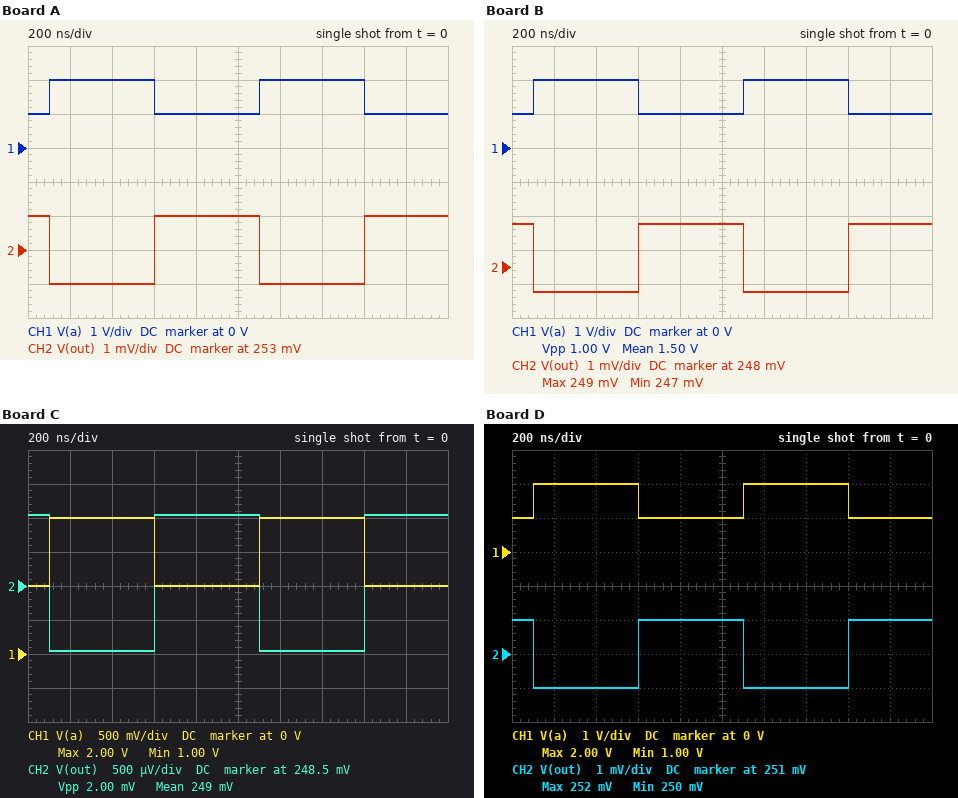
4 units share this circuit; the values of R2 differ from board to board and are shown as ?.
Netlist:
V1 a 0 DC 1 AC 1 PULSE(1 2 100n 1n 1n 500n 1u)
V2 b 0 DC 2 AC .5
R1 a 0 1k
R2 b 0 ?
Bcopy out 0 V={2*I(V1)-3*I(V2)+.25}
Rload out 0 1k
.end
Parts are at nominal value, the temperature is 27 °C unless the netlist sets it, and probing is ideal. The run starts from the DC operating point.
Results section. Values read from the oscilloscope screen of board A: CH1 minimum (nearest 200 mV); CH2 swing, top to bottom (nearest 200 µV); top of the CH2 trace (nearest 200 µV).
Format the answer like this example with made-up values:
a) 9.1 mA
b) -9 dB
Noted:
a) 1.0 V
b) 2.0 mV
c) 254.0 mV
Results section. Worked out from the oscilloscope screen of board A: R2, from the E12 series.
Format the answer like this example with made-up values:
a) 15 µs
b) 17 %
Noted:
a) 1 kΩ
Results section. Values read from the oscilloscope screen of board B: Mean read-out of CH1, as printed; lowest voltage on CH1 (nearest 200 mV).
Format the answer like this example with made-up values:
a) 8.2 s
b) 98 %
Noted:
a) 1.50 V
b) 1.0 V
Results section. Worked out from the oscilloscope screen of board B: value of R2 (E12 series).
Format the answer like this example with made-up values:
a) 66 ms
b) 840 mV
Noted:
a) 4.7 kΩ
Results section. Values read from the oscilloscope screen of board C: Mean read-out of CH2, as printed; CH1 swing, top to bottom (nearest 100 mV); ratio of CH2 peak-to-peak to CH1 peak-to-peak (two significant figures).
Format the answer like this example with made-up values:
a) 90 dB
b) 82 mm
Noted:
a) 249 mV
b) 1.0 V
c) 0.0020
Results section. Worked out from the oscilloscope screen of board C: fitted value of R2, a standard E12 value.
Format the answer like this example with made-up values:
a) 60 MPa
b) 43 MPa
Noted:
a) 3.9 kΩ
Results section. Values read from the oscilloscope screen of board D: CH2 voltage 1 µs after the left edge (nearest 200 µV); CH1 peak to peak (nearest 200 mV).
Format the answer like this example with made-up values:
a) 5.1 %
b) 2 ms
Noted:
a) 252.0 mV
b) 1.0 V
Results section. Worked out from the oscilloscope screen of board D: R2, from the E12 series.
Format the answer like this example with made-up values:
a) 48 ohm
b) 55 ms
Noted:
a) 1.5 kΩ
